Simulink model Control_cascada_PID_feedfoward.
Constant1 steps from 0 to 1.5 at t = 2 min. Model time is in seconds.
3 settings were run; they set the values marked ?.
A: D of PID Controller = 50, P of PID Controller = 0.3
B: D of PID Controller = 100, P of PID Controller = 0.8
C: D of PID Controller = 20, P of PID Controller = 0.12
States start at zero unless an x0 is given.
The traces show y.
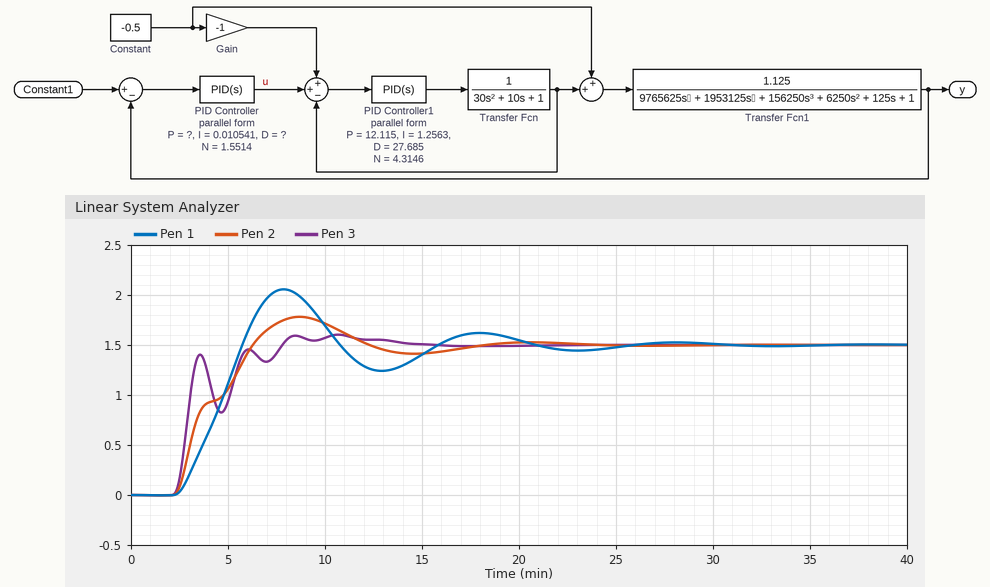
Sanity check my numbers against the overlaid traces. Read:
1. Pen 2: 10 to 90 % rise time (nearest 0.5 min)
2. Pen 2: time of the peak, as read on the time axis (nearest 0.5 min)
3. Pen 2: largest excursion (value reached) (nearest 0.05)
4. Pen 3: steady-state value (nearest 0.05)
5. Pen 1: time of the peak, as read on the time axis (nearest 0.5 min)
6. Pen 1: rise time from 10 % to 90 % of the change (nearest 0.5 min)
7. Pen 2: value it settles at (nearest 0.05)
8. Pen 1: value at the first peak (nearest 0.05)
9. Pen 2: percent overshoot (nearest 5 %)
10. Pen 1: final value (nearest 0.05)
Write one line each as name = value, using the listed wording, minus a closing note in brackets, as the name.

Pen 2: 10 to 90 % rise time = 3.0 min
Pen 2: time of the peak, as read on the time axis = 8.5 min
Pen 2: largest excursion (value reached) = 1.80
Pen 3: steady-state value = 1.50
Pen 1: time of the peak, as read on the time axis = 8.0 min
Pen 1: rise time from 10 % to 90 % of the change = 2.5 min
Pen 2: value it settles at = 1.50
Pen 1: value at the first peak = 2.05
Pen 2: percent overshoot = 20 %
Pen 1: final value = 1.50
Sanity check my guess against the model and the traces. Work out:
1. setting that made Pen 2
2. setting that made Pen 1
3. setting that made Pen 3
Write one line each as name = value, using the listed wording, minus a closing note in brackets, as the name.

setting that made Pen 2 = A
setting that made Pen 1 = C
setting that made Pen 3 = B
